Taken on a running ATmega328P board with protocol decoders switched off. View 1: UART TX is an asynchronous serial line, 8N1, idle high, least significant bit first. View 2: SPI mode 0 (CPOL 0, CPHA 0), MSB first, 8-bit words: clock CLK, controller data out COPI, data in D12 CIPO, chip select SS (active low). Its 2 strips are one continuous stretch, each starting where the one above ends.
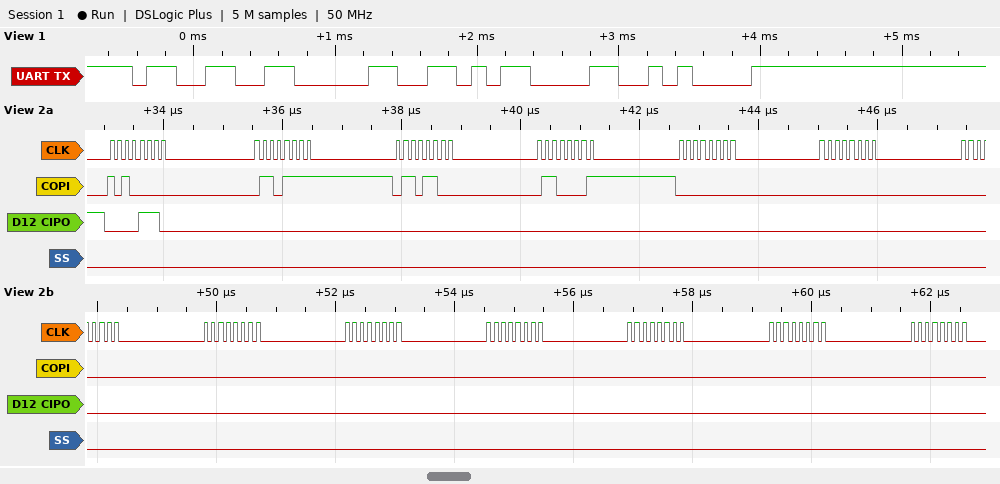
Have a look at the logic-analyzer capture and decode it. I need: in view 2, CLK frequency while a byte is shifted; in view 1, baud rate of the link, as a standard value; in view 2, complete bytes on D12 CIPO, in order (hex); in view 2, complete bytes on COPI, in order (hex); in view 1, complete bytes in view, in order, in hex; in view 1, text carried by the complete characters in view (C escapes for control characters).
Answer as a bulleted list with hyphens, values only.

- 8 MHz
- 9600 baud
- 0x0E 0x00 0x00 0x00 0x00 0x00 0x00 0x00 0x00 0x00 0x00 0x00 0x00
- 0xA0 0x6F 0x6C 0x61 0x00 0x00 0x00 0x00 0x00 0x00 0x00 0x00 0x00
- 0x33 0x30 0x0D 0x0A
- "30\r\n"
